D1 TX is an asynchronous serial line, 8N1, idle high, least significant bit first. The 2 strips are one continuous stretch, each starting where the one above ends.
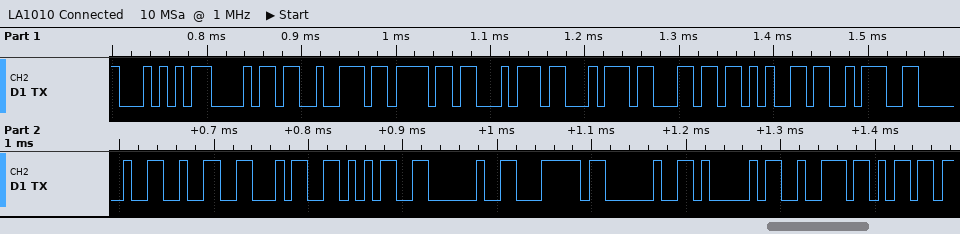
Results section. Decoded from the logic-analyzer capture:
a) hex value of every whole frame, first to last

54 68 72 6F 74 74 6C 65 3A 20 32 34 35 20 7C 20 41 72 6D
